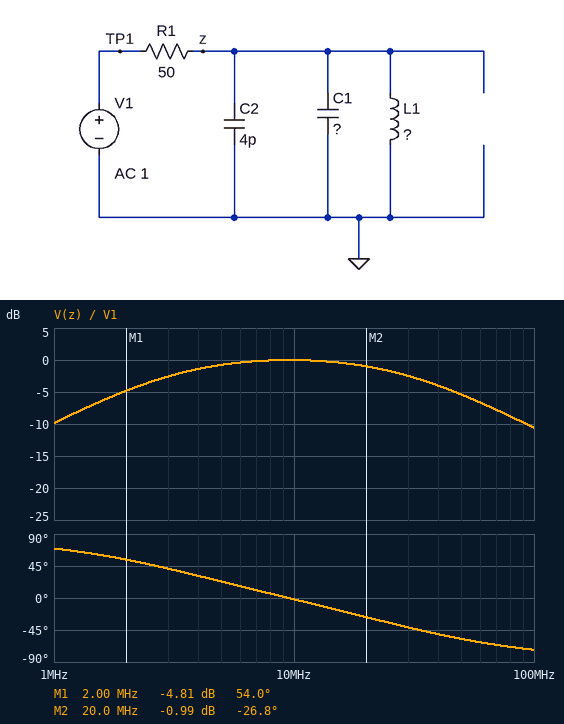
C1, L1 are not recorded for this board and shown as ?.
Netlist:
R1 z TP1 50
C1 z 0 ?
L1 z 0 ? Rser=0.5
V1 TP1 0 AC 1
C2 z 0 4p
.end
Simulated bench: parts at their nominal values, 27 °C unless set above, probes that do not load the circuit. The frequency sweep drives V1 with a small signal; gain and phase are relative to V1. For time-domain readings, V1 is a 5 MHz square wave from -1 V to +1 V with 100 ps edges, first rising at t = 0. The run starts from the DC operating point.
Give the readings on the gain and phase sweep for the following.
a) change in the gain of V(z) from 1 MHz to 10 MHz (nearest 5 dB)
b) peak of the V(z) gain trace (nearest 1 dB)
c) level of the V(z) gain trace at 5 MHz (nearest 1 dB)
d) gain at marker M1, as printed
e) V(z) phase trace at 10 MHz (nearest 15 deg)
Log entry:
10 dB
0 dB
-1 dB
-4.81 dB
0 deg
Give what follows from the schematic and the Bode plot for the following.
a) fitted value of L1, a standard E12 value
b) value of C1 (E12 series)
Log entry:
2.7 µH
100 pF
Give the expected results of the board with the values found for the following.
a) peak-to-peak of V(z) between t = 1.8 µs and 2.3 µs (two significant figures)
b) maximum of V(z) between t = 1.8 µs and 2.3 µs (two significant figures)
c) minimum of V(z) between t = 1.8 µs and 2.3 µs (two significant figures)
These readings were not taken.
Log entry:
2.9 V
1.5 V
-1.5 V
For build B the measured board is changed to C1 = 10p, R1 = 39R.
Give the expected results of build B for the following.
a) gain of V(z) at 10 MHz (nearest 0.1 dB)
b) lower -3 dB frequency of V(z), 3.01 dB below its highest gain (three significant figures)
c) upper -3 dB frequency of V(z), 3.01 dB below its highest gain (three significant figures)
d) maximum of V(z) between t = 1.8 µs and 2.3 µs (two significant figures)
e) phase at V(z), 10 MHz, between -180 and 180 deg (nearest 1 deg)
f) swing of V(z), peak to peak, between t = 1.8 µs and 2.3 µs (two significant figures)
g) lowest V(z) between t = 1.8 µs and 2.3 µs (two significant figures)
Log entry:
-0.2 dB
2.31 MHz
294 MHz
1.6 V
11 deg
3.1 V
-1.6 V
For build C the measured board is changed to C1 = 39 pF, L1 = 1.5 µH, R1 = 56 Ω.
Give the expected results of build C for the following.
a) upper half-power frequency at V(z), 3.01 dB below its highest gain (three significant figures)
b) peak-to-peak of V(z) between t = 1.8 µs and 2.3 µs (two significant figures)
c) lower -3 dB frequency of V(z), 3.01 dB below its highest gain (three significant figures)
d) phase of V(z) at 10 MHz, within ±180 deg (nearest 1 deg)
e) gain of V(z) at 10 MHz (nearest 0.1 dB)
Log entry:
71.7 MHz
3.3 V
5.53 MHz
24 deg
-0.8 dB
